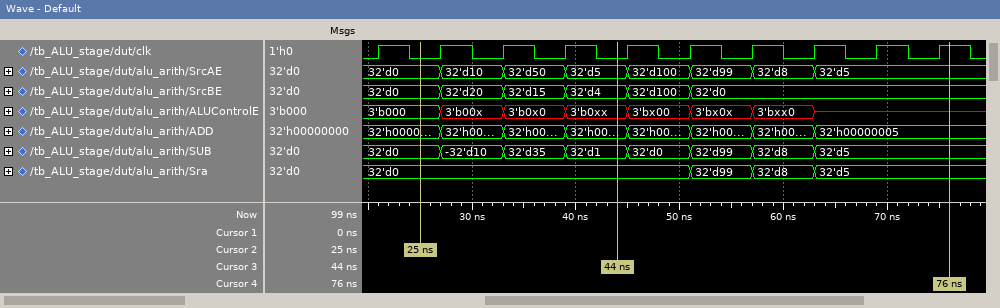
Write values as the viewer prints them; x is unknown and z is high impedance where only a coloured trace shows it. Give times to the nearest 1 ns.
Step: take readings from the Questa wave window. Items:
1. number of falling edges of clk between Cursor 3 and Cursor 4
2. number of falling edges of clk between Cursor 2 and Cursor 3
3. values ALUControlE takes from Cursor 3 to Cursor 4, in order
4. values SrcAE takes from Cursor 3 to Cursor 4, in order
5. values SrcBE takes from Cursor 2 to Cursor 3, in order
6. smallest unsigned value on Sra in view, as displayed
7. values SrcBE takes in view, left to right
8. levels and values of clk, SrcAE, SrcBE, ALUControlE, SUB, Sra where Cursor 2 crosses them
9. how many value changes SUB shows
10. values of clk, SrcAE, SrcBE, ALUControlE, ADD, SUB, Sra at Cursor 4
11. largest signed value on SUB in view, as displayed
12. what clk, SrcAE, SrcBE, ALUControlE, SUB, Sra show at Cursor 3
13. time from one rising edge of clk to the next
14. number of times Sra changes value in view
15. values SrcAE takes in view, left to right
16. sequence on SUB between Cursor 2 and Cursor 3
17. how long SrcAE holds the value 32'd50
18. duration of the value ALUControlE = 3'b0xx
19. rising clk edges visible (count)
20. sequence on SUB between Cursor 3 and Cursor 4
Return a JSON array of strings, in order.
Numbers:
["5", "3", "3'b0xx, 3'bx00, 3'bx0x, 3'bxx0, x", "32'd5, 32'd100, 32'd99, 32'd8, 32'd5", "32'd0, 32'd20, 32'd15, 32'd4", "32'd0", "32'd0, 32'd20, 32'd15, 32'd4, 32'd100, 32'd0", "clk=0, SrcAE=32'd0, SrcBE=32'd0, ALUControlE=3'b000, SUB=32'd0, Sra=32'd0", "7", "clk=1, SrcAE=32'd5, SrcBE=32'd0, ALUControlE=x, ADD=32'h00000005, SUB=32'd5, Sra=32'd5", "32'd99", "clk=0, SrcAE=32'd5, SrcBE=32'd4, ALUControlE=3'b0xx, SUB=32'd1, Sra=32'd0", "6 ns", "3", "32'd0, 32'd10, 32'd50, 32'd5, 32'd100, 32'd99, 32'd8, 32'd5", "32'd0, -32'd10, 32'd35, 32'd1", "6 ns", "6 ns", "10", "32'd1, 32'd0, 32'd99, 32'd8, 32'd5"]
